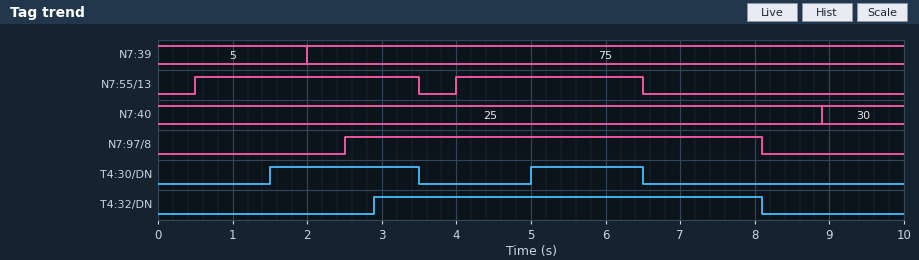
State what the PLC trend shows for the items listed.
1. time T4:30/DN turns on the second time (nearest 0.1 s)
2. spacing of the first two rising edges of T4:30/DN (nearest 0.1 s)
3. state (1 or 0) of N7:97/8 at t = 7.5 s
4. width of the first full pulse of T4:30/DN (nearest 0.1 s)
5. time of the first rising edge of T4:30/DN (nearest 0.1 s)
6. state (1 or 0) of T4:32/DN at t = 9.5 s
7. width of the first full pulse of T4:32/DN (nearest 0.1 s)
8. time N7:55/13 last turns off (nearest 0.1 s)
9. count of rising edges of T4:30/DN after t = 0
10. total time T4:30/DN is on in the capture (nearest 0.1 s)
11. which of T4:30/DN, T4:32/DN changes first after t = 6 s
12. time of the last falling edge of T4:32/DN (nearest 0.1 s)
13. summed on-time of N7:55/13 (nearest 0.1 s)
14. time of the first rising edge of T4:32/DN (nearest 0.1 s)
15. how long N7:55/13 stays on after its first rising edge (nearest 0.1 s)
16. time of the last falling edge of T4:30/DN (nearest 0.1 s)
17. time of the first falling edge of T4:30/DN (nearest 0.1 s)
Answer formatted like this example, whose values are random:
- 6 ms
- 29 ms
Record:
- 5.0 s
- 3.5 s
- 1
- 2.0 s
- 1.5 s
- 0
- 5.2 s
- 6.5 s
- 2
- 3.5 s
- T4:30/DN
- 8.1 s
- 5.5 s
- 2.9 s
- 3.0 s
- 6.5 s
- 3.5 s
